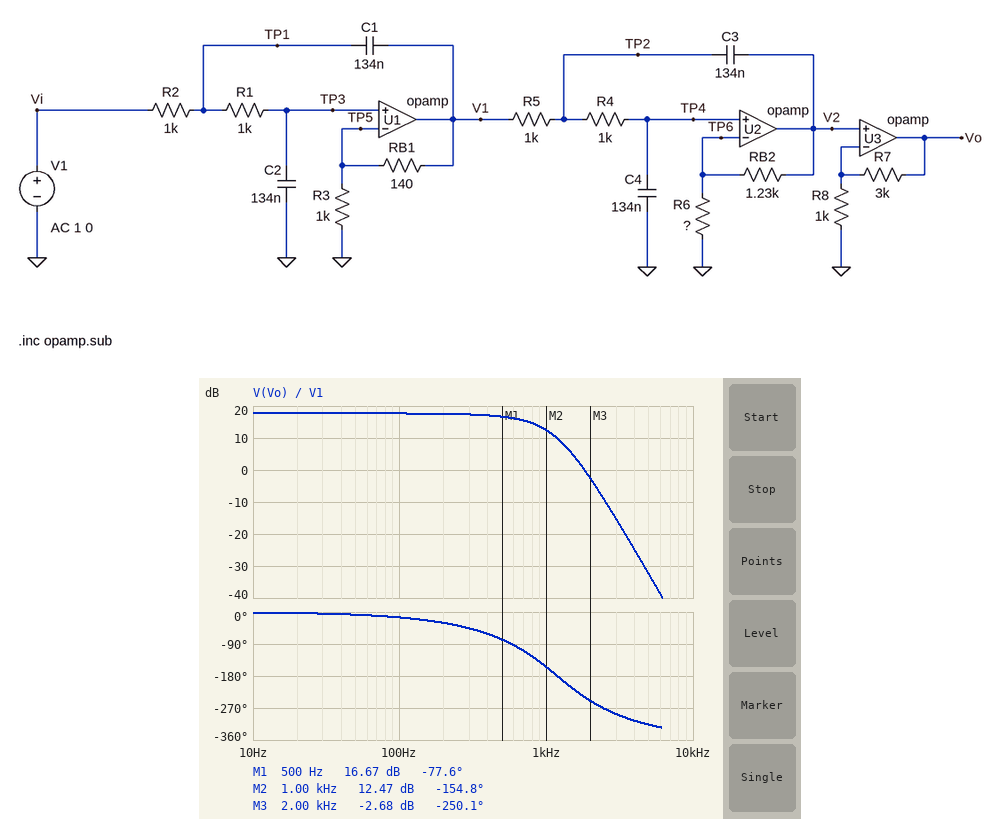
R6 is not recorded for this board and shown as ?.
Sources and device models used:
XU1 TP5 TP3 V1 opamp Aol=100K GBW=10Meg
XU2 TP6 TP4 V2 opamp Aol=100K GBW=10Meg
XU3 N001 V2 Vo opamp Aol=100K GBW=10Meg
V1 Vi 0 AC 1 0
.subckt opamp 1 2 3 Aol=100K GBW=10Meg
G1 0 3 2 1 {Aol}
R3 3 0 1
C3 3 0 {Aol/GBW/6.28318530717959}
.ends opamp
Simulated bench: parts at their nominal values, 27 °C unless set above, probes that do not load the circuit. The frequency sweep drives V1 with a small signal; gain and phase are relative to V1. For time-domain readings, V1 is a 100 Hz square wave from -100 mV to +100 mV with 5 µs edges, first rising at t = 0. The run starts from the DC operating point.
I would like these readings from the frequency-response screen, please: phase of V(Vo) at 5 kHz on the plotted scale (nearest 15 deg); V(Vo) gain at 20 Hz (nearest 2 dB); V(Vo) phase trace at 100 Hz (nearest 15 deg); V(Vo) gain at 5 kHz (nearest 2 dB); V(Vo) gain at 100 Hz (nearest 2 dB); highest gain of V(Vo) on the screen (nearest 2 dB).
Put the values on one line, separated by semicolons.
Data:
-315 deg; 18 dB; -15 deg; -32 dB; 18 dB; 18 dB
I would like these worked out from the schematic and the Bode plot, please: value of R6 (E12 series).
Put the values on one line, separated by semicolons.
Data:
1.8 kΩ
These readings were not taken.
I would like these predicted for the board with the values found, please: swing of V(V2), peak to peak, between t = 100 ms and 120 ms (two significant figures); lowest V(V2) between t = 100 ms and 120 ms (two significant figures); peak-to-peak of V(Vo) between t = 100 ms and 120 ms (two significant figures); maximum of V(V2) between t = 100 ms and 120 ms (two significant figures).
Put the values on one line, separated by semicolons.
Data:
400 mV; -200 mV; 1.6 V; 200 mV
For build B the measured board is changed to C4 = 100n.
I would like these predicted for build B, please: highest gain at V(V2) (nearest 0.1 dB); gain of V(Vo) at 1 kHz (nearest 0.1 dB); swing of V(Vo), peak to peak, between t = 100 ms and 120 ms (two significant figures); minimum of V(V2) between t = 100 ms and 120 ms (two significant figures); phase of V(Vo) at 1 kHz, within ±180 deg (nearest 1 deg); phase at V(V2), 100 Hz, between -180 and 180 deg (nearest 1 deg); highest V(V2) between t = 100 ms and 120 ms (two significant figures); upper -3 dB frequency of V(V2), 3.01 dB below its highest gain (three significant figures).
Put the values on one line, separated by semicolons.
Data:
5.7 dB; 15.3 dB; 1.7 V; -210 mV; -135 deg; -13 deg; 210 mV; 1.08 kHz
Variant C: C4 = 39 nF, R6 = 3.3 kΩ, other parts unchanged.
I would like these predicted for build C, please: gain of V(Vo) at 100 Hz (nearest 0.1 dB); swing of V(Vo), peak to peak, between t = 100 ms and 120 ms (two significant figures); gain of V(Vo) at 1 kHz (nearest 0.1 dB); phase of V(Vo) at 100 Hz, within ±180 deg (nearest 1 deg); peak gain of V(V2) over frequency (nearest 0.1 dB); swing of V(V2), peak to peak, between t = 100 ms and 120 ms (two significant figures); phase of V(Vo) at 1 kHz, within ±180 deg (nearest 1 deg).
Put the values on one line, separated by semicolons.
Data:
15.9 dB; 1.3 V; 13.7 dB; -10 deg; 3.9 dB; 330 mV; -92 deg
